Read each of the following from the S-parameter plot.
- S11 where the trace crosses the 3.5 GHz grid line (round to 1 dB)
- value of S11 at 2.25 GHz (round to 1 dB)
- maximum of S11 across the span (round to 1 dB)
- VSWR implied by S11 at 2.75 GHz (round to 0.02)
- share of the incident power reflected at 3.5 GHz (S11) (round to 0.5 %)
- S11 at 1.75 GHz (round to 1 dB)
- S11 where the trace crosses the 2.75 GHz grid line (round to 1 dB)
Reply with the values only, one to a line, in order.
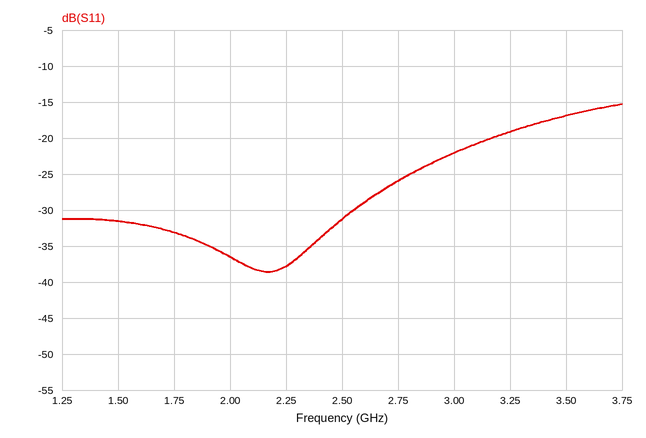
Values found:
-17 dB
-38 dB
-15 dB
1.10
2.0 %
-33 dB
-26 dB
